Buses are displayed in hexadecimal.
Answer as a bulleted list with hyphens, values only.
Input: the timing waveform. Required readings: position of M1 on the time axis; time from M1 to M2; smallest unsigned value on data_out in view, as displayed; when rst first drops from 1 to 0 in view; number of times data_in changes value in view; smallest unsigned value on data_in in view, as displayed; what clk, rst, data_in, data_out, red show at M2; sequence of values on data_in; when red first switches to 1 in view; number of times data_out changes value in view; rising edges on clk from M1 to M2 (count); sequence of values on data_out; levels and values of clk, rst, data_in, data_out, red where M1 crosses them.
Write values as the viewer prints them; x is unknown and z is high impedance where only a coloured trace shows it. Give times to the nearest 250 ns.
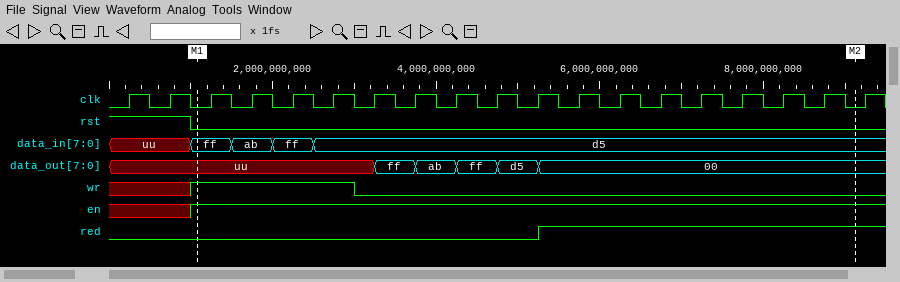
- 1000 ns
- 8000 ns
- 00
- 1000 ns
- 4
- ab
- clk=0, rst=0, data_in=d5, data_out=00, red=1
- uu, ff, ab, ff, d5
- 5250 ns
- 5
- 16
- uu, ff, ab, ff, d5, 00
- clk=0, rst=0, data_in=ff, data_out=uu, red=0
